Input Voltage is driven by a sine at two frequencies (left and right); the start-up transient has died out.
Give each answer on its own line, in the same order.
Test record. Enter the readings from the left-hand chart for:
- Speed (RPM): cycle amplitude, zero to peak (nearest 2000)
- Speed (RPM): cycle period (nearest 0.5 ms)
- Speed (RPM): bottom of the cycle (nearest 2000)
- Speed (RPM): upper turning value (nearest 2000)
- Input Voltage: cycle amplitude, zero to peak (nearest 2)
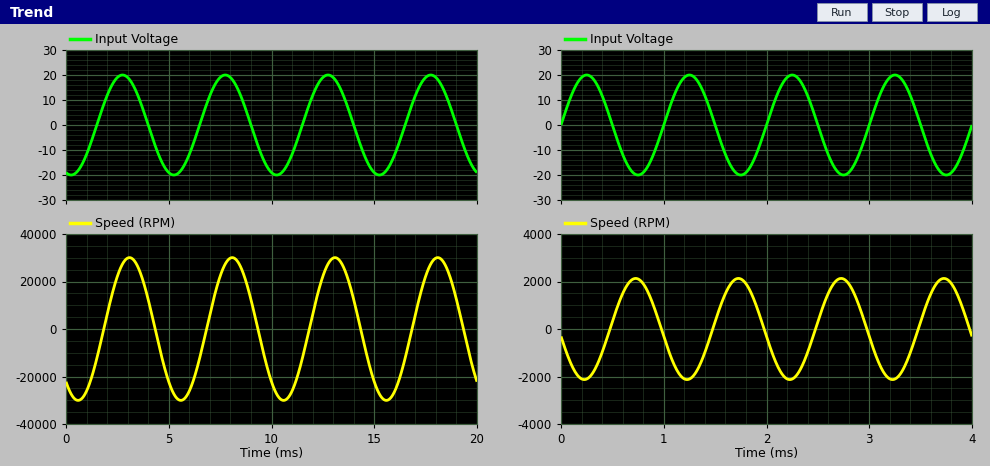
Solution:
30000
5.0 ms
-30000
30000
20
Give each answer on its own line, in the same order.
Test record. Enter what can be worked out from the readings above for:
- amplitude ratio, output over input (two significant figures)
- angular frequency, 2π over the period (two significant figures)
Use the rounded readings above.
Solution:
1500
1.3 rad/ms
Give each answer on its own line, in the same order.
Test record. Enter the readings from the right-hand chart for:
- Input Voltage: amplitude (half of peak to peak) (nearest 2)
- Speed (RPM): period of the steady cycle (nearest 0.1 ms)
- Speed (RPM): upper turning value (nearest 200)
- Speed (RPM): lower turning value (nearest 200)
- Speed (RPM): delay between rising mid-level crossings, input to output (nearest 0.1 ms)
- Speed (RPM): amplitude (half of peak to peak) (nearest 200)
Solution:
20
1.0 ms
2200
-2200
0.5 ms
2200
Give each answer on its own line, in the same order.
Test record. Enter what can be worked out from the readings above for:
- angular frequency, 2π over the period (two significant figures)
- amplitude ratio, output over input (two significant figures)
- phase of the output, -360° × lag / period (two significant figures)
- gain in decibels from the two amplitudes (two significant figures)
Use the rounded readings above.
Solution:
6.3 rad/ms
110
-180°
41 dB
